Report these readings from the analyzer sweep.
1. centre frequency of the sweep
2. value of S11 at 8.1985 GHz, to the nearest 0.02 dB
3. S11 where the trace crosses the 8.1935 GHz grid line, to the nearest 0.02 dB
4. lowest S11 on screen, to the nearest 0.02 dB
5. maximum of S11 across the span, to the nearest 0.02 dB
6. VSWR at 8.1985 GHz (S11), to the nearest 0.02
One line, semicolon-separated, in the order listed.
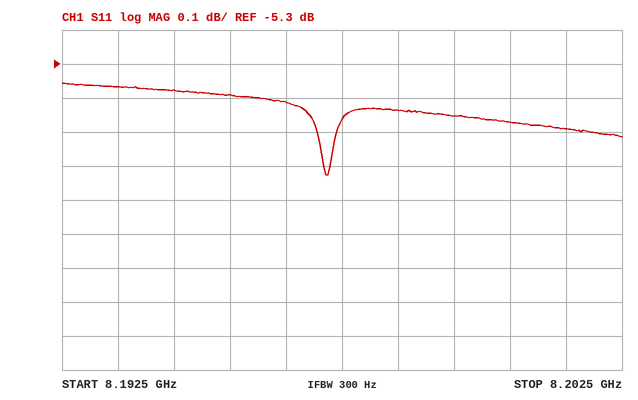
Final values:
8.1975 GHz; -5.44 dB; -5.36 dB; -5.62 dB; -5.36 dB; 3.30
